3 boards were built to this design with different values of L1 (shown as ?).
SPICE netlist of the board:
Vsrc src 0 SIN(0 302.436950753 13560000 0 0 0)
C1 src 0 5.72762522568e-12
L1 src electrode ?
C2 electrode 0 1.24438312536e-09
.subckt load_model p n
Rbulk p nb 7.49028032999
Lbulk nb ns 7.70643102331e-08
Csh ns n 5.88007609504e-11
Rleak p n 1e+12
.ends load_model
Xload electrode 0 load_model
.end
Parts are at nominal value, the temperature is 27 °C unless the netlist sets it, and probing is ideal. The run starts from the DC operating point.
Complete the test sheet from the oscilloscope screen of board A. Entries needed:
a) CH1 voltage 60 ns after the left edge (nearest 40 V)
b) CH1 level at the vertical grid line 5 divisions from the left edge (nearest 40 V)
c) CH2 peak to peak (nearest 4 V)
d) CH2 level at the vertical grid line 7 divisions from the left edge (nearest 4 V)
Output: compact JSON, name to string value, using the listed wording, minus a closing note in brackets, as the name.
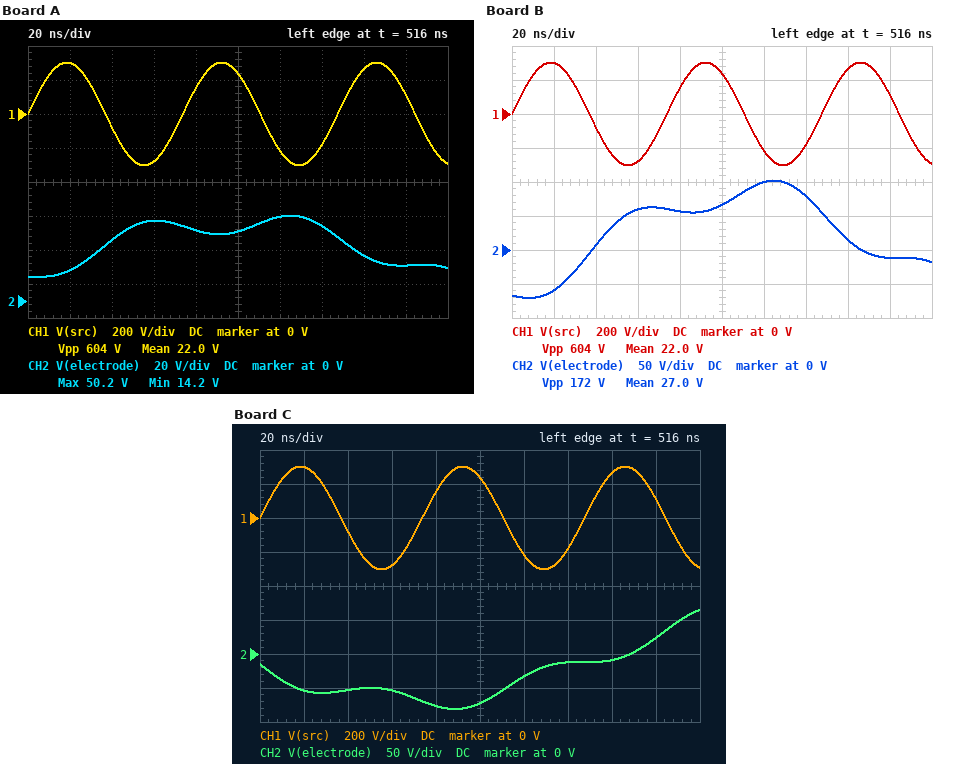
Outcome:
{"CH1 voltage 60 ns after the left edge": "-280 V", "CH1 level at the vertical grid line 5 divisions from the left edge": "240 V", "CH2 peak to peak": "36 V", "CH2 level at the vertical grid line 7 divisions from the left edge": "44 V"}
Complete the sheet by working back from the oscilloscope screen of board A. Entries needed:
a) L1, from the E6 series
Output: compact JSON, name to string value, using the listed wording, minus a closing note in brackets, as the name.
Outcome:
{"L1, from the E6 series": "4.7 µH"}
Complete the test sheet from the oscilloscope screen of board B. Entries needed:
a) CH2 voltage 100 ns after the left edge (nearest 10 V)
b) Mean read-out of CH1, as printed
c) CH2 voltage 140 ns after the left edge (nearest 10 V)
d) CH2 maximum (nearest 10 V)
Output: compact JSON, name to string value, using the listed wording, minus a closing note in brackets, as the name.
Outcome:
{"CH2 voltage 100 ns after the left edge": "70 V", "Mean read-out of CH1, as printed": "22.0 V", "CH2 voltage 140 ns after the left edge": "80 V", "CH2 maximum": "100 V"}
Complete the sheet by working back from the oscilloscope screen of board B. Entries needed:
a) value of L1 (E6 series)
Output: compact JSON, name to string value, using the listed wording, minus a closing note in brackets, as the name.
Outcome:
{"value of L1": "1.5 µH"}
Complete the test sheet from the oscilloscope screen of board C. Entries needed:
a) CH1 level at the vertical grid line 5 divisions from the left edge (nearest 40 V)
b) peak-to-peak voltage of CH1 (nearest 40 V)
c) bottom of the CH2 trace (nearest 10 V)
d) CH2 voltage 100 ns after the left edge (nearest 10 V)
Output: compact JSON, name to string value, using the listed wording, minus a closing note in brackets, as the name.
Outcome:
{"CH1 level at the vertical grid line 5 divisions from the left edge": "240 V", "peak-to-peak voltage of CH1": "600 V", "bottom of the CH2 trace": "-80 V", "CH2 voltage 100 ns after the left edge": "-70 V"}
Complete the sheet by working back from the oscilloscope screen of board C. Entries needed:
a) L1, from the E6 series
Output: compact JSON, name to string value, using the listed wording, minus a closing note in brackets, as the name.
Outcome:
{"L1, from the E6 series": "2.2 µH"}
